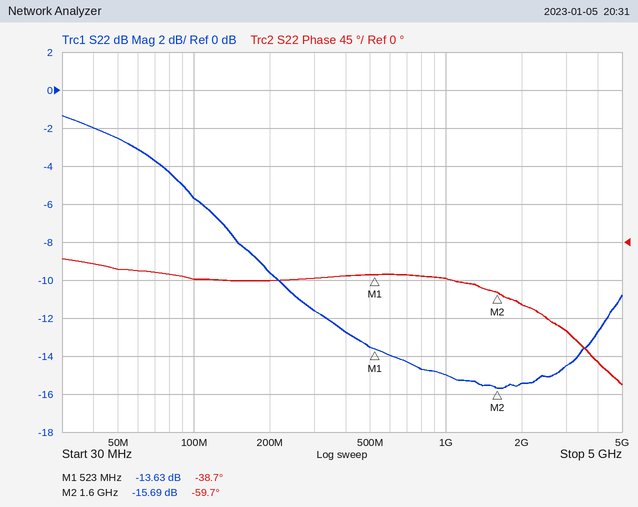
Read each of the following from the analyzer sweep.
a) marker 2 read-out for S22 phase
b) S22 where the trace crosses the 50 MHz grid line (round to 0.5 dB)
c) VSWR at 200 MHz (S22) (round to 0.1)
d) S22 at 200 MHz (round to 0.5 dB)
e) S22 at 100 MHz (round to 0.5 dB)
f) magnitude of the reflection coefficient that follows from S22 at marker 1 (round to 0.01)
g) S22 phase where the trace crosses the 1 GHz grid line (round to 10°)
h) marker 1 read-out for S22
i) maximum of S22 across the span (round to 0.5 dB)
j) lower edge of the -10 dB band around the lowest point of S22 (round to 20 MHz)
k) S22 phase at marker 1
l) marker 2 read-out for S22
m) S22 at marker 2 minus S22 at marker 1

-59.7°
-2.5 dB
2.0
-9.5 dB
-5.5 dB
0.21
-40°
-13.63 dB
-1.5 dB
220 MHz
-38.7°
-15.69 dB
-2.06 dB
